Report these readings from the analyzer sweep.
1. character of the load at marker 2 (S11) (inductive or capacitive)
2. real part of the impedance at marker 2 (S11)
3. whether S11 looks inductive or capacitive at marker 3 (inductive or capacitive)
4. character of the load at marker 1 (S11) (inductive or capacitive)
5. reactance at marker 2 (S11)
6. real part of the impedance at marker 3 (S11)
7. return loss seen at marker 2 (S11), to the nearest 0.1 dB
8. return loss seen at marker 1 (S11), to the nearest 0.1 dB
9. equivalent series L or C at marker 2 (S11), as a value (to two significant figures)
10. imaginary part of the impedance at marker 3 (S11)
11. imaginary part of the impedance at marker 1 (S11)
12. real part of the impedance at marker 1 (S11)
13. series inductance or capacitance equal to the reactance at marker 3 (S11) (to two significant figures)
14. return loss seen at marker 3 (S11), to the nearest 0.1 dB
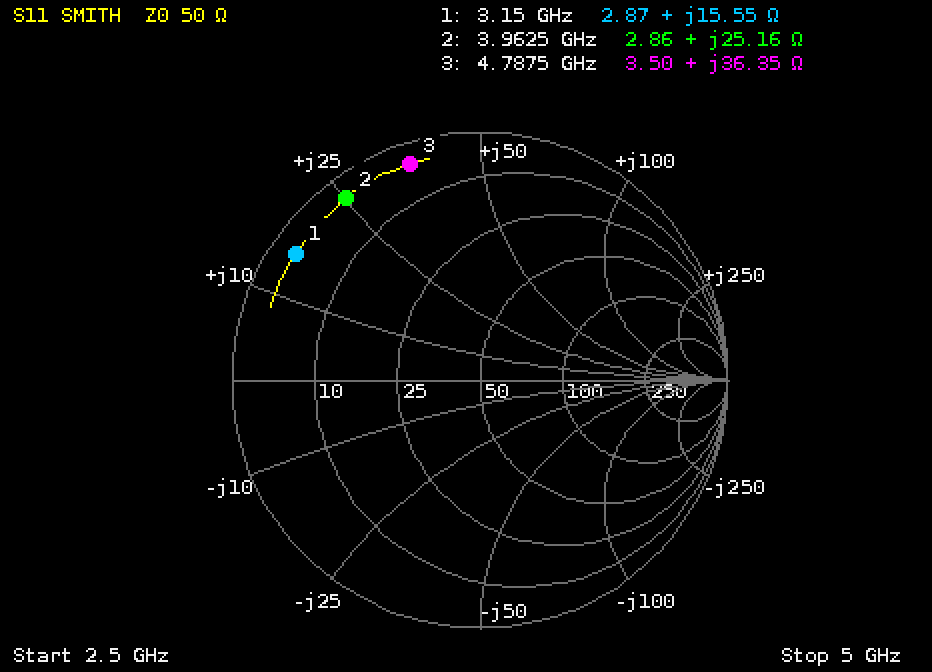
inductive
2.86 Ω
inductive
inductive
+25.16 Ω
3.50 Ω
0.8 dB
0.9 dB
1.0 nH
+36.35 Ω
+15.55 Ω
2.87 Ω
1.2 nH
0.8 dB
